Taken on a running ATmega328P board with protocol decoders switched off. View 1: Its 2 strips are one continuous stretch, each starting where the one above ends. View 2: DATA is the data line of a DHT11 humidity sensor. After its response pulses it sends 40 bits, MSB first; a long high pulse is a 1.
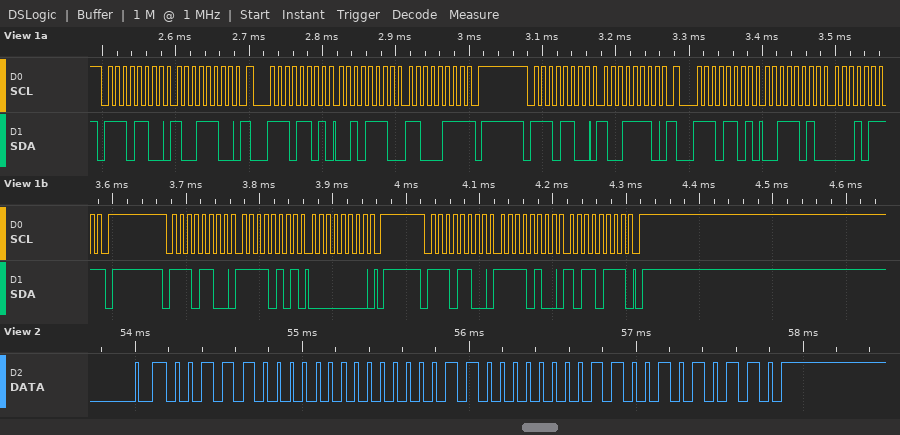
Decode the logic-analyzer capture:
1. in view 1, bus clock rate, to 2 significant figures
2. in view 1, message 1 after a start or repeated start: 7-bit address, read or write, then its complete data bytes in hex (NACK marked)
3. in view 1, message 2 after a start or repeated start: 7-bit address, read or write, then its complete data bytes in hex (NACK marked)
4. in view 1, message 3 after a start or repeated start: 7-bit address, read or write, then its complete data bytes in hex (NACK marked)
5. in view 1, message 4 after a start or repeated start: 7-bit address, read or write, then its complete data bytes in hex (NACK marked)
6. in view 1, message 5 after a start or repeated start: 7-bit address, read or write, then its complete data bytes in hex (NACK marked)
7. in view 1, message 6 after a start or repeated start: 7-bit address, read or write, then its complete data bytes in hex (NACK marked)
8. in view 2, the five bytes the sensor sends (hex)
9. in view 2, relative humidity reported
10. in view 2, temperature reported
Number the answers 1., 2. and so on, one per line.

1. 100 kHz
2. 0x76 write: 9C
3. 0x76 read: 2E C7 NACK
4. 0x76 write: 9E
5. 0x76 read: 3A 17 NACK
6. 0x76 write: F5 00
7. 0x76 write: F4 B7
8. 38 00 18 06 56
9. 56 %
10. 24.6 °C
